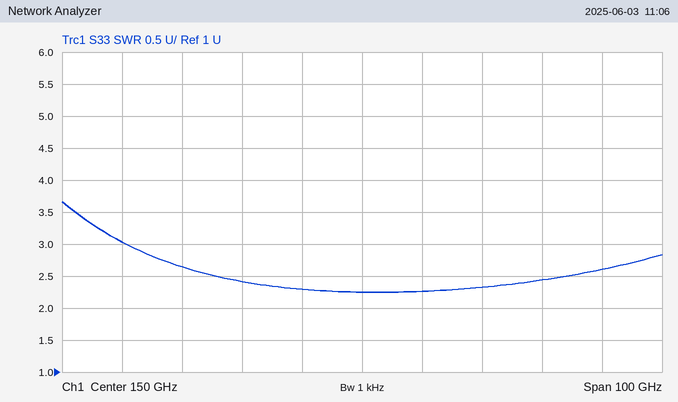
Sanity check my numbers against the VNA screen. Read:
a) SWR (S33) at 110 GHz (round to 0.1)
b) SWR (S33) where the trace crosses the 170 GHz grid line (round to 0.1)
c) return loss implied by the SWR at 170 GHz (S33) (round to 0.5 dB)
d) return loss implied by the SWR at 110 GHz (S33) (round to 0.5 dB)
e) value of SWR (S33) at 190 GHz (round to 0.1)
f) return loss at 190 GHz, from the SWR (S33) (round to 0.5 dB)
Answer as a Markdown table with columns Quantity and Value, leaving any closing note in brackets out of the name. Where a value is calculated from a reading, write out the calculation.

| Quantity | Value |
|---|---|
| SWR (S33) at 110 GHz | 3.0 |
| SWR (S33) where the trace crosses the 170 GHz grid line | 2.3 |
| return loss implied by the SWR at 170 GHz (S33) | −20 log10((2.3 − 1)/(2.3 + 1)) ≈ 8.09 dB, so 8.0 dB to the nearest 0.5 dB |
| return loss implied by the SWR at 110 GHz (S33) | −20 log10((3 − 1)/(3 + 1)) ≈ 6.0 dB |
| value of SWR (S33) at 190 GHz | 2.6 |
| return loss at 190 GHz, from the SWR (S33) | −20 log10((2.6 − 1)/(2.6 + 1)) ≈ 7.0 dB |
